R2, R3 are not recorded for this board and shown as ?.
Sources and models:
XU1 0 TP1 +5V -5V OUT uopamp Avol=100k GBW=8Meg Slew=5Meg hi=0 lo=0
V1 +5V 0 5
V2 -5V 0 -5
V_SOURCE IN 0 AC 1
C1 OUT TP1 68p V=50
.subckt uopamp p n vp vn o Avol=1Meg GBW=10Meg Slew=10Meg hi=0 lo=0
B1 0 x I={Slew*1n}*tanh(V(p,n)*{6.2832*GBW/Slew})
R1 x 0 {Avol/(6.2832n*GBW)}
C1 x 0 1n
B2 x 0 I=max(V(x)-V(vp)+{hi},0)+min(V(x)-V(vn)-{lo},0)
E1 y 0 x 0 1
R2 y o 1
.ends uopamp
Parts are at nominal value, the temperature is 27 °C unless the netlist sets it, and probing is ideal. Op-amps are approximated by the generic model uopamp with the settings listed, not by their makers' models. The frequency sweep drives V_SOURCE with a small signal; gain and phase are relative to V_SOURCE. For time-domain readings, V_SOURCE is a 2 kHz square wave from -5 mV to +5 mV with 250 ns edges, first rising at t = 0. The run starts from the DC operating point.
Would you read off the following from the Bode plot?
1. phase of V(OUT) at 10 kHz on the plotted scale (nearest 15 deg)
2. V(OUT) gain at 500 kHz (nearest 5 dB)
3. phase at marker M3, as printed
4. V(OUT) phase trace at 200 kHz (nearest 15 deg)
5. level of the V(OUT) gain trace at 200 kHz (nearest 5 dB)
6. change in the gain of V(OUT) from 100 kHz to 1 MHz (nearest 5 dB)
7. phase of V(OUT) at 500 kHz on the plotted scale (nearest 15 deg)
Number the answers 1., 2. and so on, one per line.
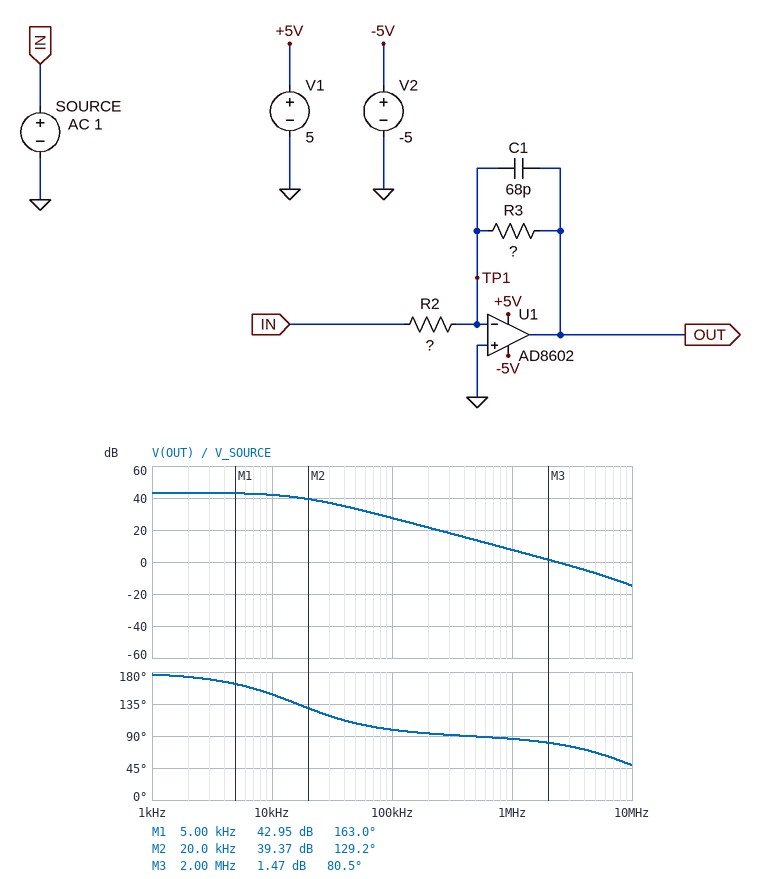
1. 150 deg
2. 15 dB
3. 80.5 deg
4. 90 deg
5. 20 dB
6. -20 dB
7. 90 deg
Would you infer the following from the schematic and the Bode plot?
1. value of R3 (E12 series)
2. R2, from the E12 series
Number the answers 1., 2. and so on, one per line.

1. 100 kΩ
2. 680 Ω
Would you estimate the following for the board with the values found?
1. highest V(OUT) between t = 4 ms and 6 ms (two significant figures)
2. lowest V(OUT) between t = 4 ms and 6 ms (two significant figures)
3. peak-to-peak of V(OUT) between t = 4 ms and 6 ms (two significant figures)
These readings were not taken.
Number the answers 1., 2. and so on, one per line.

1. 730 mV
2. -730 mV
3. 1.5 V
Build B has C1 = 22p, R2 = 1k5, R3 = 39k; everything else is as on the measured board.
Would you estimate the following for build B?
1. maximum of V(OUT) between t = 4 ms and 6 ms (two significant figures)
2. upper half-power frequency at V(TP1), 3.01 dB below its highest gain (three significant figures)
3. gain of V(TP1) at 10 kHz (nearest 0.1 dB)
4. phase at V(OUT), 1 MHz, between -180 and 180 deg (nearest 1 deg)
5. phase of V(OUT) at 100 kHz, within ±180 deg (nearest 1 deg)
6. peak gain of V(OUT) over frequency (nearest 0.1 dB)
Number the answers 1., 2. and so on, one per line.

1. 130 mV
2. 13.1 MHz
3. -29.8 dB
4. 92 deg
5. 139 deg
6. 28.3 dB
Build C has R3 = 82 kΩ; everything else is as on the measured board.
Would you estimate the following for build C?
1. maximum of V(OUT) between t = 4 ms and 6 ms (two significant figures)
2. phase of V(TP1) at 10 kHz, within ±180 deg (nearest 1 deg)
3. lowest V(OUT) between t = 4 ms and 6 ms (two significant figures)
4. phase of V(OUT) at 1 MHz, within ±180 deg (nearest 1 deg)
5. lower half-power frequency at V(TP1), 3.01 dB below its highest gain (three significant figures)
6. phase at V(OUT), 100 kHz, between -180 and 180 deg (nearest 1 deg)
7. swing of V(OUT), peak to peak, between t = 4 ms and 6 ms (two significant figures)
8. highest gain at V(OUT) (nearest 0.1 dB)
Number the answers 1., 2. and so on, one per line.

1. 600 mV
2. 63 deg
3. -600 mV
4. 86 deg
5. 19.9 kHz
6. 101 deg
7. 1.2 V
8. 41.6 dB
